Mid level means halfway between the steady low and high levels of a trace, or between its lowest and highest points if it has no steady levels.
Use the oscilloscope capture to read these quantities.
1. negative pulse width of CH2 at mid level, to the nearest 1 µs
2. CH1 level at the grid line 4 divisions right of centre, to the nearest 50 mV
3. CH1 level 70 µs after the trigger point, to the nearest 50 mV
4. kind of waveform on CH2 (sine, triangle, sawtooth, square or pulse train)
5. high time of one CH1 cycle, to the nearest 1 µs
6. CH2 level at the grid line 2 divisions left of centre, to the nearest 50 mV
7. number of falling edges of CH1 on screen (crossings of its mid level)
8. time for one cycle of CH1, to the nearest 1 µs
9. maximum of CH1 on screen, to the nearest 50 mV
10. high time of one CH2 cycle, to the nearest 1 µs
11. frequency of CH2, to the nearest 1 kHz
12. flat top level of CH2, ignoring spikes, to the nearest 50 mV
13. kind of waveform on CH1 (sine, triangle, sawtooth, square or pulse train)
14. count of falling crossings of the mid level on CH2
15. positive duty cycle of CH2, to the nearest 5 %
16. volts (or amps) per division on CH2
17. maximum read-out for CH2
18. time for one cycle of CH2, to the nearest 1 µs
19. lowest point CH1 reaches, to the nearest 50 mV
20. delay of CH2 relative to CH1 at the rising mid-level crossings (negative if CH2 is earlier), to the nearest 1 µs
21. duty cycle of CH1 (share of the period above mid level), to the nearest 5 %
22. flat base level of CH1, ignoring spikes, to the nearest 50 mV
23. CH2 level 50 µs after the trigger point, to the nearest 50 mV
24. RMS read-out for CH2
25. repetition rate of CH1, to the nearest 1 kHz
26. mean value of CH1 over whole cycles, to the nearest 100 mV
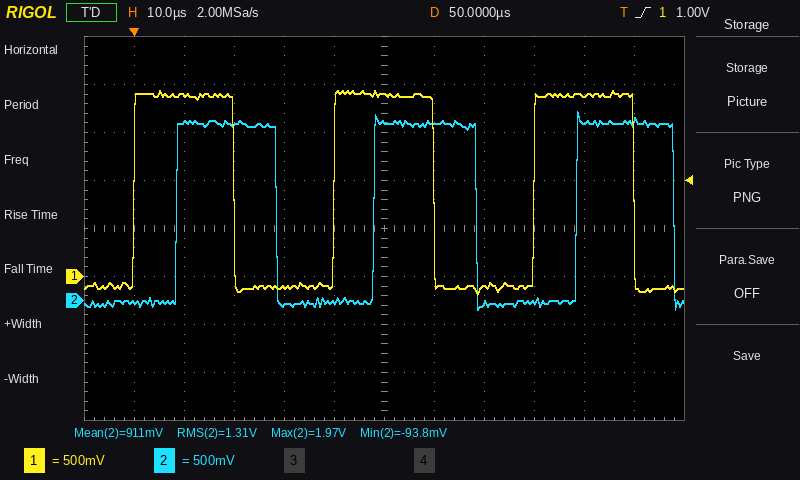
20 µs
1.90 V
-100 mV
square
20 µs
-50 mV
3
40 µs
1.95 V
20 µs
25 kHz
1.85 V
square
3
50 %
500 mV
1.97 V
40 µs
-200 mV
+8 µs
50 %
-100 mV
1.85 V
1.31 V
25 kHz
900 mV
